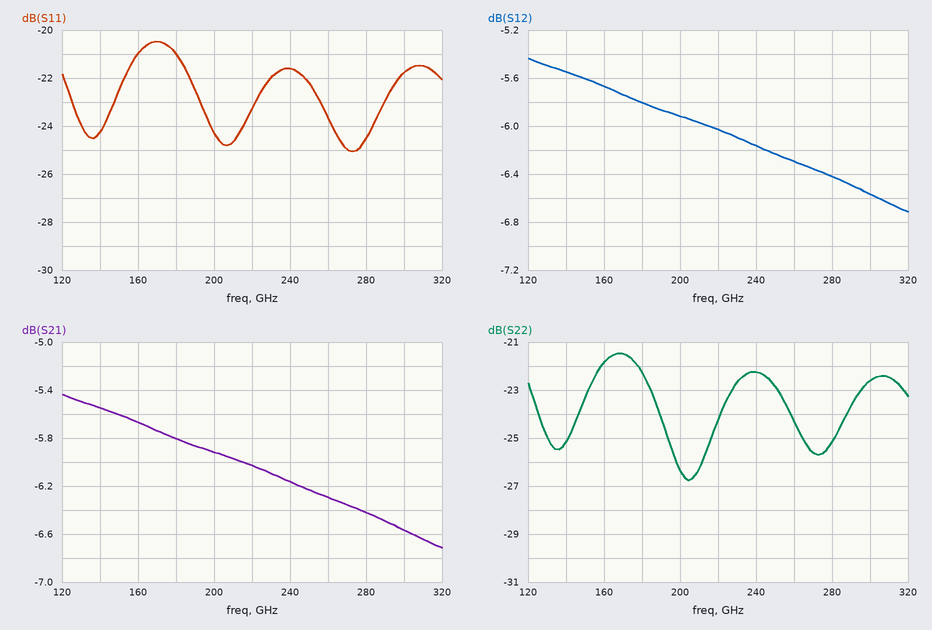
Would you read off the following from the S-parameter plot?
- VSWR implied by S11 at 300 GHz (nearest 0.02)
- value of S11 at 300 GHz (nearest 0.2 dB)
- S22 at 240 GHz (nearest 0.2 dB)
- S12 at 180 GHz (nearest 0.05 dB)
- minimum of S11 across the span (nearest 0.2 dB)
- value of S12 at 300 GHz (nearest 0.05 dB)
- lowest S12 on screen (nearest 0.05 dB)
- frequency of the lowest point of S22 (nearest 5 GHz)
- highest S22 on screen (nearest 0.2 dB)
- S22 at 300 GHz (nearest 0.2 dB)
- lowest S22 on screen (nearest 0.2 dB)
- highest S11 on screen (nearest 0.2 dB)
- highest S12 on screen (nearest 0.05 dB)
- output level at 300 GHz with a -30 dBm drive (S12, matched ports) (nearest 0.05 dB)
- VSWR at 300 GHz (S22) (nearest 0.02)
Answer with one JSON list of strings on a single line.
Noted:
["1.18", "-21.8 dB", "-22.2 dB", "-5.80 dB", "-25.0 dB", "-6.55 dB", "-6.70 dB", "205 GHz", "-21.4 dB", "-22.6 dB", "-26.8 dB", "-20.4 dB", "-5.45 dB", "-36.55 dBm", "1.16"]
